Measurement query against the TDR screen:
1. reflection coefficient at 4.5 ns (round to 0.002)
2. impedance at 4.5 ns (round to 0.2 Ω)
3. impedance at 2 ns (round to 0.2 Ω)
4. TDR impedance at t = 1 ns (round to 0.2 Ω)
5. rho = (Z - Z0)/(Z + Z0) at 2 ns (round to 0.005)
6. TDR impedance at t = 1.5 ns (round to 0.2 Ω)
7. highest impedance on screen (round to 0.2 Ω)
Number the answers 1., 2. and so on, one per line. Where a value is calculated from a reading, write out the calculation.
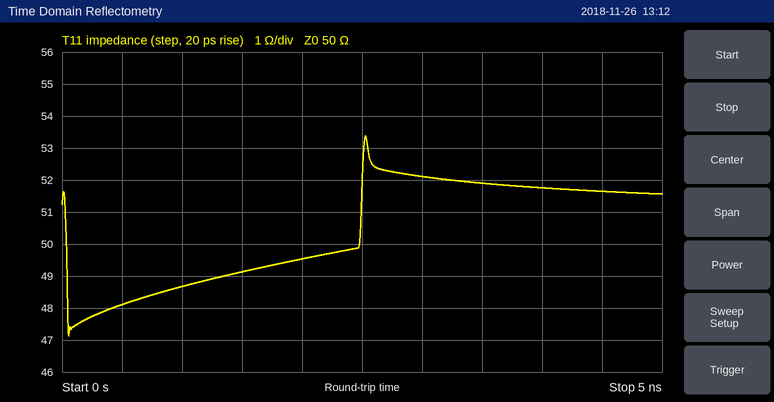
1. (51.6 − 50)/(51.6 + 50) ≈ +0.016
2. 51.6 Ω
3. 49.6 Ω
4. 48.6 Ω
5. (49.6 − 50)/(49.6 + 50) ≈ -0.00402, so -0.005 to the nearest 0.005
6. 49.2 Ω
7. 53.4 Ω
